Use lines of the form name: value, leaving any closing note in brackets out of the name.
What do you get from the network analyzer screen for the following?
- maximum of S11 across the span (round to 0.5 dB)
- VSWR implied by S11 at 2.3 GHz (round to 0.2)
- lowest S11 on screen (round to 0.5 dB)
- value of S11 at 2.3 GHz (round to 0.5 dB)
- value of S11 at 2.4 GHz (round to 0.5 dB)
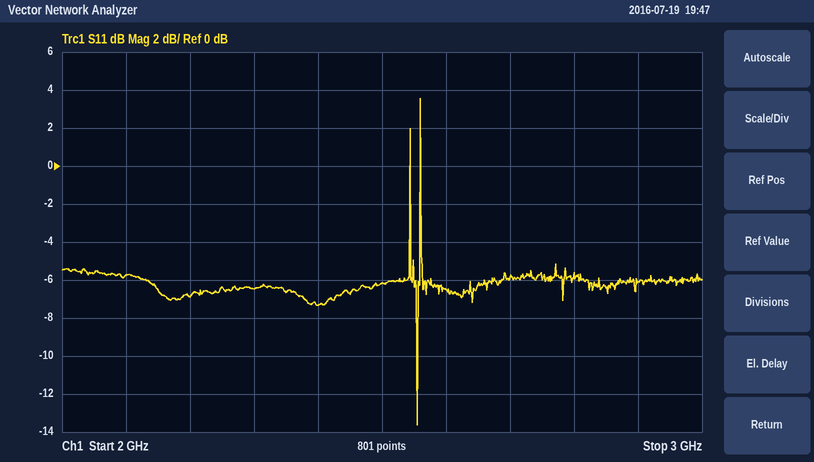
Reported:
maximum of S11 across the span: 3.5 dB
VSWR implied by S11 at 2.3 GHz: 2.8
lowest S11 on screen: -13.5 dB
value of S11 at 2.3 GHz: -6.5 dB
value of S11 at 2.4 GHz: -7.5 dB
